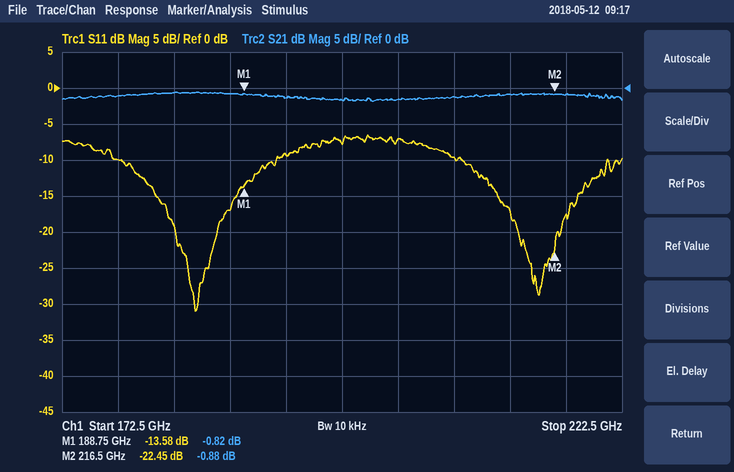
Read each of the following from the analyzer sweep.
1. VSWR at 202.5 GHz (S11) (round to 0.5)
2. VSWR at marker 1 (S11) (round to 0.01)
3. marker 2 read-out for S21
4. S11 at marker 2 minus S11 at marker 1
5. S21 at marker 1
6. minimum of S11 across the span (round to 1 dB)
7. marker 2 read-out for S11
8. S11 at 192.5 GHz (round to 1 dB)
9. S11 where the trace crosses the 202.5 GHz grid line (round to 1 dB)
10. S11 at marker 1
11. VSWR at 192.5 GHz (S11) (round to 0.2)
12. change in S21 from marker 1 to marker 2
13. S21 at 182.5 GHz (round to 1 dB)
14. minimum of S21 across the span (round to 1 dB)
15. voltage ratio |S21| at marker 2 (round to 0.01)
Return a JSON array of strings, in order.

["2.5", "1.53", "-0.88 dB", "-8.87 dB", "-0.82 dB", "-31 dB", "-22.45 dB", "-9 dB", "-7 dB", "-13.58 dB", "2.0", "-0.06 dB", "-1 dB", "-2 dB", "0.90"]
